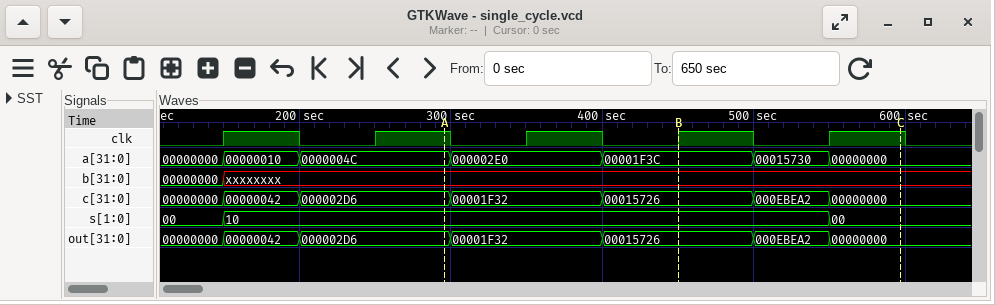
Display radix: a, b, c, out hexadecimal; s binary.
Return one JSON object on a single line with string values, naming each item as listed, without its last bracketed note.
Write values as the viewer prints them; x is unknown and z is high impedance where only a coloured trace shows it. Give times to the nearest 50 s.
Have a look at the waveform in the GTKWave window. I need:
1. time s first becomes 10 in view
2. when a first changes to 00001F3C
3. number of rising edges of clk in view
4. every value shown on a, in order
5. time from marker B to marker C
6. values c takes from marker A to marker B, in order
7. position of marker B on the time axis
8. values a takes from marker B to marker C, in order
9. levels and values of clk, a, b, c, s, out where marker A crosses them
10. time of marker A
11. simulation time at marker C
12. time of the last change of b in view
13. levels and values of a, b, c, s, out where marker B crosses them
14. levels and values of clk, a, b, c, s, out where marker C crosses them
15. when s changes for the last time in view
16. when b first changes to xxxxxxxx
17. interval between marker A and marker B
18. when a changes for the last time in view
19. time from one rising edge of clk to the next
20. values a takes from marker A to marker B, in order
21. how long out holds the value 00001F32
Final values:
{"time s first becomes 10 in view": "150 s", "when a first changes to 00001F3C": "400 s", "number of rising edges of clk in view": "5", "every value shown on a, in order": "00000000, 00000010, 0000004C, 000002E0, 00001F3C, 00015730, 00000000", "time from marker B to marker C": "150 s", "values c takes from marker A to marker B, in order": "000002D6, 00001F32, 00015726", "position of marker B on the time axis": "450 s", "values a takes from marker B to marker C, in order": "00001F3C, 00015730, 00000000", "levels and values of clk, a, b, c, s, out where marker A crosses them": "clk=1, a=0000004C, b=xxxxxxxx, c=000002D6, s=10, out=000002D6", "time of marker A": "300 s", "simulation time at marker C": "600 s", "time of the last change of b in view": "150 s", "levels and values of a, b, c, s, out where marker B crosses them": "a=00001F3C, b=xxxxxxxx, c=00015726, s=10, out=00015726", "levels and values of clk, a, b, c, s, out where marker C crosses them": "clk=1, a=00000000, b=xxxxxxxx, c=00000000, s=00, out=00000000", "when s changes for the last time in view": "550 s", "when b first changes to xxxxxxxx": "150 s", "interval between marker A and marker B": "150 s", "when a changes for the last time in view": "550 s", "time from one rising edge of clk to the next": "100 s", "values a takes from marker A to marker B, in order": "0000004C, 000002E0, 00001F3C", "how long out holds the value 00001F32": "100 s"}
